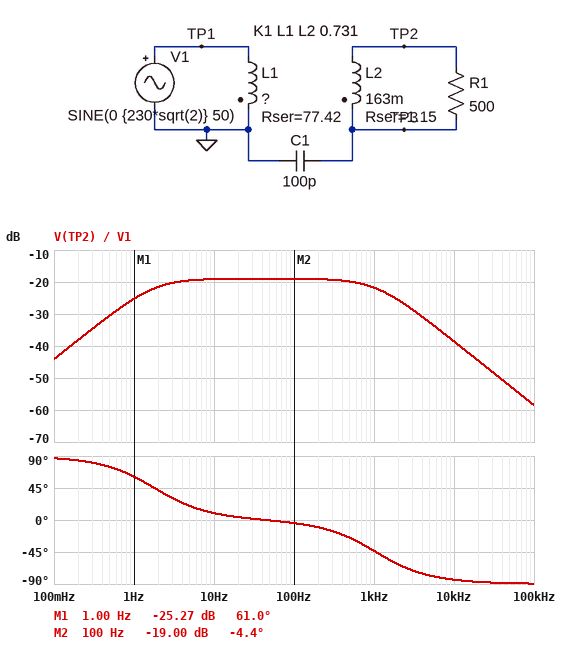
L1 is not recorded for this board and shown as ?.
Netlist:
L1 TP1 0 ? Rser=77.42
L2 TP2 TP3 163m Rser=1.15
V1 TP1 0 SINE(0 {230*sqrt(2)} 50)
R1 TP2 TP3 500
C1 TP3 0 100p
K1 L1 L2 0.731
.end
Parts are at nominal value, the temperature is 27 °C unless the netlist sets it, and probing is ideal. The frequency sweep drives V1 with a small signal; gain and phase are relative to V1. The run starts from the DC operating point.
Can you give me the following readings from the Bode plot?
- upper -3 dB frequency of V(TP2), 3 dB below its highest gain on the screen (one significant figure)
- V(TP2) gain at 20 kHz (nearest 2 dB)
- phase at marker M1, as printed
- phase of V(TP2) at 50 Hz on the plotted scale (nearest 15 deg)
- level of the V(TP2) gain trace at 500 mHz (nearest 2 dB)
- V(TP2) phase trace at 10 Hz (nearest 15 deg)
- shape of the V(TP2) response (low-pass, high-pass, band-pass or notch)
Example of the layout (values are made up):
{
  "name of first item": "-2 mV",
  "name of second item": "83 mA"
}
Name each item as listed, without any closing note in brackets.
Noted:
{
  "upper -3 dB frequency of V(TP2), 3 dB below its highest gain on the screen": "1 kHz",
  "V(TP2) gain at 20 kHz": "-44 dB",
  "phase at marker M1, as printed": "61.0 deg",
  "phase of V(TP2) at 50 Hz on the plotted scale": "0 deg",
  "level of the V(TP2) gain trace at 500 mHz": "-30 dB",
  "V(TP2) phase trace at 10 Hz": "15 deg",
  "shape of the V(TP2) response": "band-pass"
}
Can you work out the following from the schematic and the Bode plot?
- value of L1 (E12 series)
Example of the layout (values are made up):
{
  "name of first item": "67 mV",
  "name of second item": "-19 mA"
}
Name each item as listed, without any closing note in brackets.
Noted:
{
  "value of L1": "6.8 H"
}
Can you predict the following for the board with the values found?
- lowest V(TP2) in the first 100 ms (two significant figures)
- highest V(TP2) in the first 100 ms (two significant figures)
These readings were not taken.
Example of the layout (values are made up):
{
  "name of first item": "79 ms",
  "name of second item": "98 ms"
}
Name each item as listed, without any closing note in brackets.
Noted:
{
  "lowest V(TP2) in the first 100 ms": "-38 V",
  "highest V(TP2) in the first 100 ms": "36 V"
}
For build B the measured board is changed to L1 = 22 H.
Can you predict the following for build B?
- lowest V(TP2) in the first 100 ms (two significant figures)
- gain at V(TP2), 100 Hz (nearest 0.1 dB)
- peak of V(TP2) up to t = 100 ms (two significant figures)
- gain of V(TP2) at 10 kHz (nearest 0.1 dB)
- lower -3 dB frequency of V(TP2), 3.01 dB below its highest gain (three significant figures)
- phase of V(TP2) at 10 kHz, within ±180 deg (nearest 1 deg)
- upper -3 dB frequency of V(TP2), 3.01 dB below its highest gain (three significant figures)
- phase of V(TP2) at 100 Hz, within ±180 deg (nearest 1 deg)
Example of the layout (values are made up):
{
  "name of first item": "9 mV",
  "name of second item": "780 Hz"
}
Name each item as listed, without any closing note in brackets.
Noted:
{
  "lowest V(TP2) in the first 100 ms": "-21 V",
  "gain at V(TP2), 100 Hz": "-24.1 dB",
  "peak of V(TP2) up to t = 100 ms": "20 V",
  "gain of V(TP2) at 10 kHz": "-43.7 dB",
  "lower -3 dB frequency of V(TP2), 3.01 dB below its highest gain": "559 mHz",
  "phase of V(TP2) at 10 kHz, within ±180 deg": "-84 deg",
  "upper -3 dB frequency of V(TP2), 3.01 dB below its highest gain": "1.05 kHz",
  "phase of V(TP2) at 100 Hz, within ±180 deg": "-5 deg"
}
